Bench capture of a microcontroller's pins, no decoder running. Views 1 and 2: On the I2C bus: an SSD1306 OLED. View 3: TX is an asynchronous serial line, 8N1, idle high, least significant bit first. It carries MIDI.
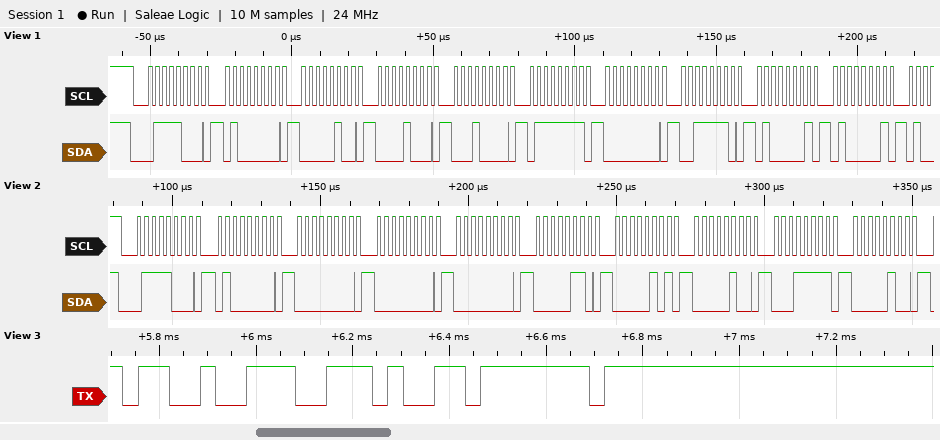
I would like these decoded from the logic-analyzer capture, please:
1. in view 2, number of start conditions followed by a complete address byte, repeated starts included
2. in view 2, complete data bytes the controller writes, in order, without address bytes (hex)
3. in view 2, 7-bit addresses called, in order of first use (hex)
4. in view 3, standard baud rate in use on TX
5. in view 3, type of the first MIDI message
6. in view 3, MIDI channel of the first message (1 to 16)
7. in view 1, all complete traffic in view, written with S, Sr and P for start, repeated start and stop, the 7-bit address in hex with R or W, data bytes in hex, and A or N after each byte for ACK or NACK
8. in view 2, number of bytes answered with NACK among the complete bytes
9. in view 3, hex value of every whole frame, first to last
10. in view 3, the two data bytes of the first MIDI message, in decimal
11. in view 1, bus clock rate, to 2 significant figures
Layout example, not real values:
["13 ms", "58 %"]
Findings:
["1", "40 00 00 00 06 05 04 1F 04", "0x3C", "31250 baud", "Note On", "4", "S 3CW A 40 A 04 A 08 A 10 A 7F A 00 A 3E A 41 A 41 A", "0", "0x93 0x2E 0x7F", "46, 127", "400 kHz"]
